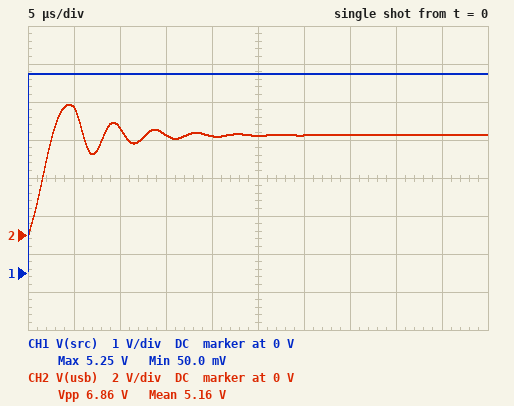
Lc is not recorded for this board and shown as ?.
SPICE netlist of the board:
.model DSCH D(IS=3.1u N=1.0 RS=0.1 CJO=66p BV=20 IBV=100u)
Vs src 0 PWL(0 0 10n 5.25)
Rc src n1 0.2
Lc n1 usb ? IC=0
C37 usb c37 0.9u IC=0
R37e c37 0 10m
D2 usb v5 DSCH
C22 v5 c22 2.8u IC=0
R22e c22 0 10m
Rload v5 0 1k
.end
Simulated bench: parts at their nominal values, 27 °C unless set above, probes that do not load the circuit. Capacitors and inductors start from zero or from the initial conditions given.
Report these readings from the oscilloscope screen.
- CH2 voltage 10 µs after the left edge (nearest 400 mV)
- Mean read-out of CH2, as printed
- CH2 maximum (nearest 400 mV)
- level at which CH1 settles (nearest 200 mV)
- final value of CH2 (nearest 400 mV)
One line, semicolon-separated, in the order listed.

5.6 V; 5.16 V; 6.8 V; 5.2 V; 5.2 V
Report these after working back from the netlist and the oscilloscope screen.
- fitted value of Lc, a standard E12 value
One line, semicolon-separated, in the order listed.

560 nH
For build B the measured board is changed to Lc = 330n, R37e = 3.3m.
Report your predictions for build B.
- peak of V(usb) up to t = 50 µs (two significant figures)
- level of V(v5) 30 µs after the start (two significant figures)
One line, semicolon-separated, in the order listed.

6.3 V; 5.9 V
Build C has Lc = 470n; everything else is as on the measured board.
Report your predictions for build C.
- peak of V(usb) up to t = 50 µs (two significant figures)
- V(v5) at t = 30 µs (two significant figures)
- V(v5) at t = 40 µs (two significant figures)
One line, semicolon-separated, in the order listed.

6.7 V; 6.3 V; 6.2 V
